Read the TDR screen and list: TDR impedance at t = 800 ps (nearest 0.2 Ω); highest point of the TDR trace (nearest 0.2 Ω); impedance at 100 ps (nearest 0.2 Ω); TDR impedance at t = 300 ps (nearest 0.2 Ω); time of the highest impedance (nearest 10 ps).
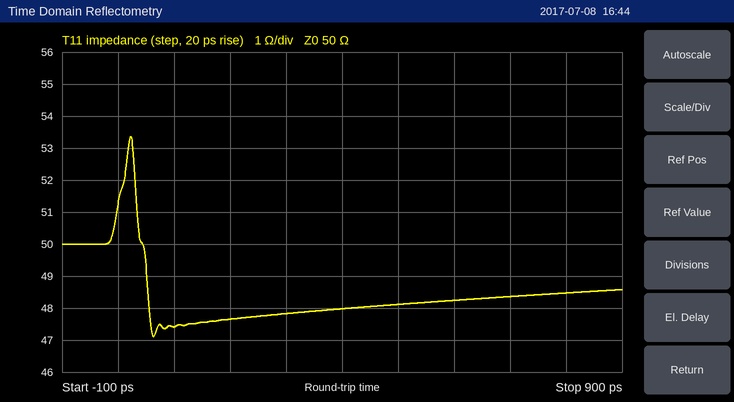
48.4 Ω
53.4 Ω
47.4 Ω
47.8 Ω
20 ps
